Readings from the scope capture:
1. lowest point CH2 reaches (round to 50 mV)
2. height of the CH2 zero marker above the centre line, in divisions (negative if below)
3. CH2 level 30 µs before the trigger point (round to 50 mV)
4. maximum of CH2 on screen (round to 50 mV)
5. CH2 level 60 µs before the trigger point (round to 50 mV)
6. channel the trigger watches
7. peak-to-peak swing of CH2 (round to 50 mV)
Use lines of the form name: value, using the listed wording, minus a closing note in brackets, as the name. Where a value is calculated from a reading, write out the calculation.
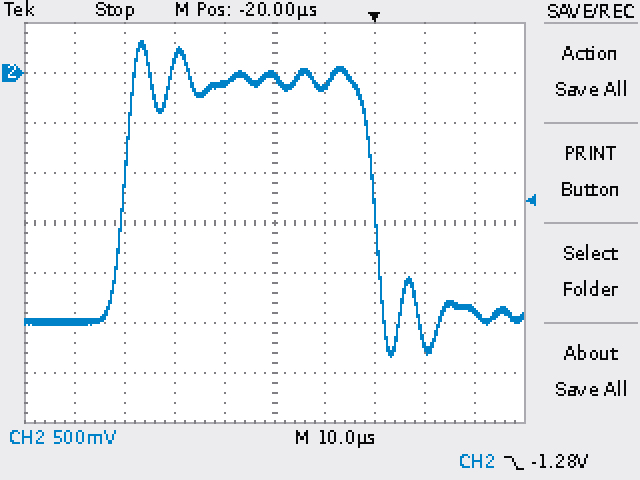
lowest point CH2 reaches: -2.85 V
height of the CH2 zero marker above the centre line, in divisions: +3.0 div
CH2 level 30 µs before the trigger point: -100 mV
maximum of CH2 on screen: 300 mV
CH2 level 60 µs before the trigger point: -2.50 V
channel the trigger watches: CH2
peak-to-peak swing of CH2: 300 mV − (-2.85 V) = 3.15 V
